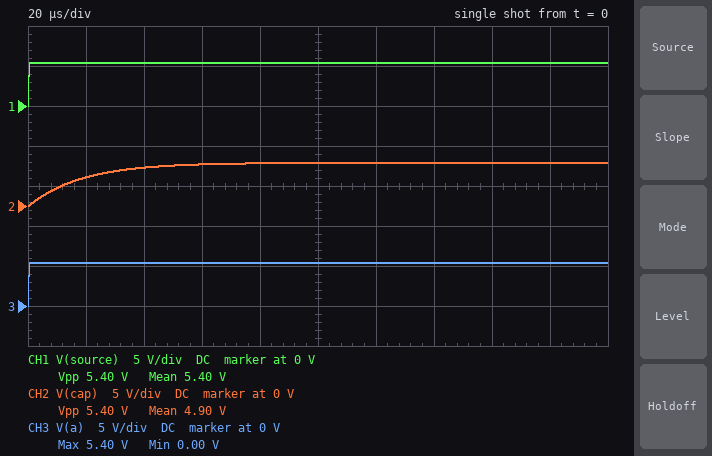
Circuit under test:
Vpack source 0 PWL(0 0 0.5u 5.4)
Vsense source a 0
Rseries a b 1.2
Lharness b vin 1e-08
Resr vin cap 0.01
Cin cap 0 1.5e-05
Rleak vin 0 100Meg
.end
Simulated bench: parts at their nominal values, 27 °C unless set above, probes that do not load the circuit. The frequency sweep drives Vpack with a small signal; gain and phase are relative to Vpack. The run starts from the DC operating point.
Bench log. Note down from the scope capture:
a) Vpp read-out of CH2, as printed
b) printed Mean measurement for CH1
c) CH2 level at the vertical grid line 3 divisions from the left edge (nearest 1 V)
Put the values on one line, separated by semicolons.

5.40 V; 5.40 V; 5 V
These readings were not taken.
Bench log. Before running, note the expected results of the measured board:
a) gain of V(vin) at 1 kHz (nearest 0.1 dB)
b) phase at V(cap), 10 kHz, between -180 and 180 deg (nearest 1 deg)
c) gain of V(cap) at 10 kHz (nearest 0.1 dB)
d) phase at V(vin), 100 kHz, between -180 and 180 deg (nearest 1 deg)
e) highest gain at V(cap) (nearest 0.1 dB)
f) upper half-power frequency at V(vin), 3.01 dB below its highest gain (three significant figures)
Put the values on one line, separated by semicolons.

-0.1 dB; -49 deg; -3.6 dB; -80 deg; 0 dB; 8.77 kHz
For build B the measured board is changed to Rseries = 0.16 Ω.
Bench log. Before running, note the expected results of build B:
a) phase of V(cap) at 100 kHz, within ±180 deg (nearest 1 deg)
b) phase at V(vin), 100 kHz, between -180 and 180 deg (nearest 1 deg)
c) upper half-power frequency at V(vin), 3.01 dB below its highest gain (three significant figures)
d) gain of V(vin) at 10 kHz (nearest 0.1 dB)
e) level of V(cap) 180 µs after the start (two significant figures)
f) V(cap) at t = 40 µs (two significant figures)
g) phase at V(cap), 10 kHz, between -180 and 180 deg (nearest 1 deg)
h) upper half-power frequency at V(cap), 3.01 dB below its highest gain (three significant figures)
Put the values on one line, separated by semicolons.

-60 deg; -54 deg; 64.1 kHz; -0.1 dB; 5.4 V; 5.4 V; -9 deg; 63.9 kHz
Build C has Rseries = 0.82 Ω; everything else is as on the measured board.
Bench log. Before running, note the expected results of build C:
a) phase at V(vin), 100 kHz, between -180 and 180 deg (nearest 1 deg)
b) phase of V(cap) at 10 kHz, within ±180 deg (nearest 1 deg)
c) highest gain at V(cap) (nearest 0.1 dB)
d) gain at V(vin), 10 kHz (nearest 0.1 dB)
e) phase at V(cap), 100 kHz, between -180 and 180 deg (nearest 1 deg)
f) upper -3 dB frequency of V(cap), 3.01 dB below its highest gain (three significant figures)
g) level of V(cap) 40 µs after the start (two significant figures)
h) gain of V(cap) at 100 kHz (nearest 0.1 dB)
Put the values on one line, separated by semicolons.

-78 deg; -38 deg; 0 dB; -2.1 dB; -83 deg; 12.8 kHz; 5.2 V; -17.9 dB
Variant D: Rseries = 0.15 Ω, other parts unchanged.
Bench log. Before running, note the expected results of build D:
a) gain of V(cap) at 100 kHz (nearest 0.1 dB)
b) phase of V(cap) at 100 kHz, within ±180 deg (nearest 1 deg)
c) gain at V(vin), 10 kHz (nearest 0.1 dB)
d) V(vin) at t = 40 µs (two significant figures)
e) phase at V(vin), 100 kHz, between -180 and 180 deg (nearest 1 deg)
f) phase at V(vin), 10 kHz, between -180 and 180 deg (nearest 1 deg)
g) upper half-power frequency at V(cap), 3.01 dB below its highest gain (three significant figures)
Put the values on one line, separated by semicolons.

-5.0 dB; -58 deg; -0.1 dB; 5.4 V; -53 deg; -8 deg; 68.1 kHz
